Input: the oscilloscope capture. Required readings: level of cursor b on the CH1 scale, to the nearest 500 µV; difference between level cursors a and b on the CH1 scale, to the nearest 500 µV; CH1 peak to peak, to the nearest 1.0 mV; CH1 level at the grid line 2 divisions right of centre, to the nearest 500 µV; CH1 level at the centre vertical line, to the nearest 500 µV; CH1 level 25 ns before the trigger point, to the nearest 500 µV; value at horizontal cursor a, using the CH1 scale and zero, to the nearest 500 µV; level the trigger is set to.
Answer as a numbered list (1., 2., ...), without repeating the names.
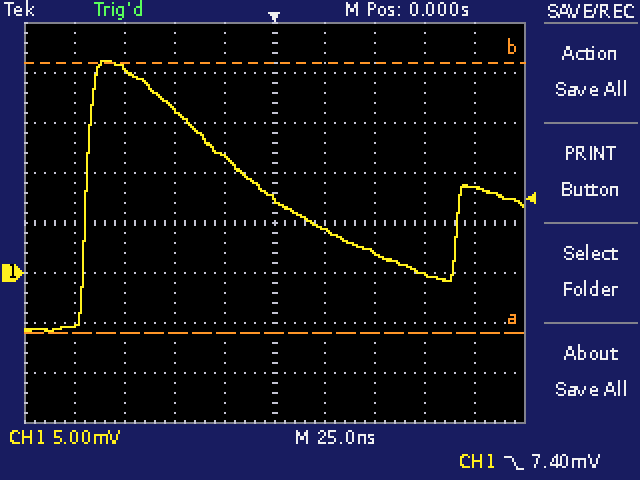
1. 21.0 mV
2. 27.0 mV
3. 27.0 mV
4. 2.0 mV
5. 7.5 mV
6. 11.5 mV
7. -6.0 mV
8. 7.40 mV
